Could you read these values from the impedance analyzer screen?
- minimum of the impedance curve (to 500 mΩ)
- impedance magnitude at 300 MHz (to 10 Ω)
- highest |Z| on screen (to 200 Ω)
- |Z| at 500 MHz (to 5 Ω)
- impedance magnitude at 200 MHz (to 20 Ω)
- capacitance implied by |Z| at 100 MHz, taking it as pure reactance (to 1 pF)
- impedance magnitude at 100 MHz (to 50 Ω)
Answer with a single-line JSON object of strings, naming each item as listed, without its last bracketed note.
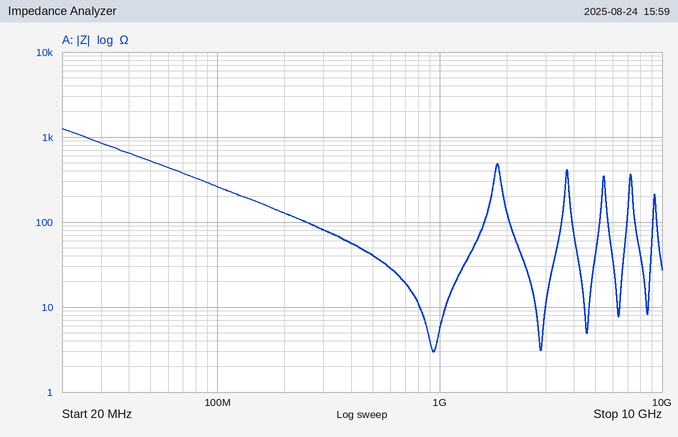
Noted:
{"minimum of the impedance curve": "3.0 Ω", "impedance magnitude at 300 MHz": "80 Ω", "highest |Z| on screen": "1.2 kΩ", "|Z| at 500 MHz": "40 Ω", "impedance magnitude at 200 MHz": "120 Ω", "capacitance implied by |Z| at 100 MHz, taking it as pure reactance": "6 pF", "impedance magnitude at 100 MHz": "250 Ω"}
